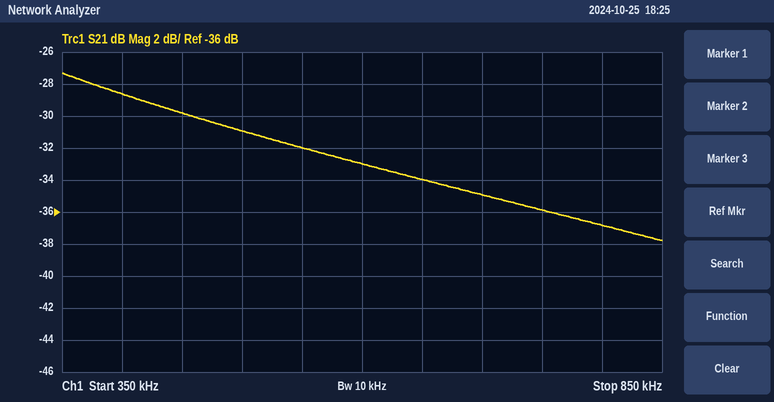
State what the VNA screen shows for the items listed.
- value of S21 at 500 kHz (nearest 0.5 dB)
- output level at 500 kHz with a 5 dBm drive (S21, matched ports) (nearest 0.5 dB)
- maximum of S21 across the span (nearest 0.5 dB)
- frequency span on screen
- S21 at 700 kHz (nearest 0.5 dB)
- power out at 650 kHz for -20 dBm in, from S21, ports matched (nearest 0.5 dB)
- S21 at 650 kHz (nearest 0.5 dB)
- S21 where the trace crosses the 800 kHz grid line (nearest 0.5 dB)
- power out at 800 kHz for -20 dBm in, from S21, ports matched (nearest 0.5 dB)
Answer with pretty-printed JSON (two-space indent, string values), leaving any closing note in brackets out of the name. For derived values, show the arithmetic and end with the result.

{
  "value of S21 at 500 kHz": "-31.0 dB",
  "output level at 500 kHz with a 5 dBm drive (S21, matched ports)": "5 dBm + (-31.0 dB) = -26.0 dBm",
  "maximum of S21 across the span": "-27.5 dB",
  "frequency span on screen": "500 kHz",
  "S21 at 700 kHz": "-35.0 dB",
  "power out at 650 kHz for -20 dBm in, from S21, ports matched": "-20 dBm + (-34.0 dB) = -54.0 dBm",
  "S21 at 650 kHz": "-34.0 dB",
  "S21 where the trace crosses the 800 kHz grid line": "-37.0 dB",
  "power out at 800 kHz for -20 dBm in, from S21, ports matched": "-20 dBm + (-37.0 dB) = -57.0 dBm"
}
